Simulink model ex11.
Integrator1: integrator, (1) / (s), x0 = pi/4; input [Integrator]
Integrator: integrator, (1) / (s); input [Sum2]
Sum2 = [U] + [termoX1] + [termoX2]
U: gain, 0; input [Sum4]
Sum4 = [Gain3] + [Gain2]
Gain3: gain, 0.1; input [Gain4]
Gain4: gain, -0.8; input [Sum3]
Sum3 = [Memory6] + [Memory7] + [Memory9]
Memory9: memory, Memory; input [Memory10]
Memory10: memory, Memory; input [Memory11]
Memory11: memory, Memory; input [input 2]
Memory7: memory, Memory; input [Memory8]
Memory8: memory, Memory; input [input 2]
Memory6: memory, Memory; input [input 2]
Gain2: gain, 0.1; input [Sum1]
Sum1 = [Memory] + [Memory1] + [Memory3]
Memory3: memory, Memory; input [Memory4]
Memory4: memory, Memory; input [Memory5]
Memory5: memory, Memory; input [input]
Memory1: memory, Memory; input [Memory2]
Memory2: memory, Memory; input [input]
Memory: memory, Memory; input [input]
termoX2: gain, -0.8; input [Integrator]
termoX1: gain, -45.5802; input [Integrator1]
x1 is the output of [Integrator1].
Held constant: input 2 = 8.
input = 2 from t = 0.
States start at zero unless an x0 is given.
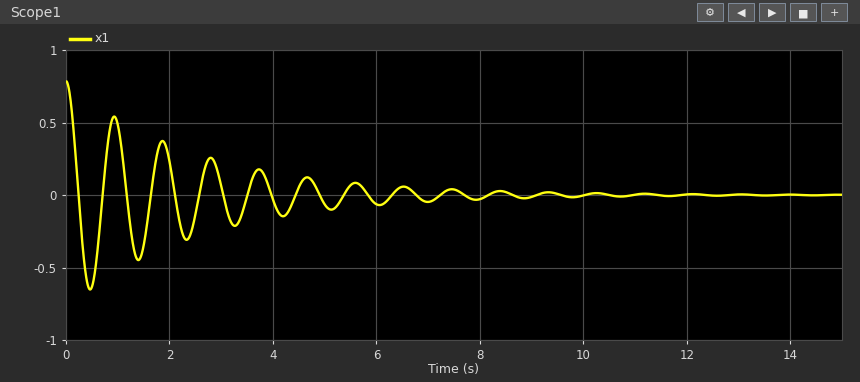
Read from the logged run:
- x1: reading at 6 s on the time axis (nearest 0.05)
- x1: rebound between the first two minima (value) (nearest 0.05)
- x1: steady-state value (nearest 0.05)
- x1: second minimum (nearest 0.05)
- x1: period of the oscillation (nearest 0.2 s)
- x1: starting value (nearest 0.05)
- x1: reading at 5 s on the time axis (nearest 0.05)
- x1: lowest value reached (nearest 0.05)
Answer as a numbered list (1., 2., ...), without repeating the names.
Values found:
1. -0.05
2. 0.55
3. 0.00
4. -0.45
5. 1.0 s
6. 0.80
7. -0.05
8. -0.65
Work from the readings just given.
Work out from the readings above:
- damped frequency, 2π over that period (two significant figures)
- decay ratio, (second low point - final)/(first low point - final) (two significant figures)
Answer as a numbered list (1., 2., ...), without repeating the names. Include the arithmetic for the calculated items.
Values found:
1. 2π / 1 = 6.3 rad/s
2. (-0.45 - 0) / (-0.65 - 0) = 0.69
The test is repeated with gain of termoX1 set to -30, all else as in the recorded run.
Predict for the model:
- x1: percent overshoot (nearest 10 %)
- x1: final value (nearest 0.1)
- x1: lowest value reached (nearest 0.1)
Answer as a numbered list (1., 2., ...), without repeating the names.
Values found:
1. 80 %
2. 0.0
3. -0.6
